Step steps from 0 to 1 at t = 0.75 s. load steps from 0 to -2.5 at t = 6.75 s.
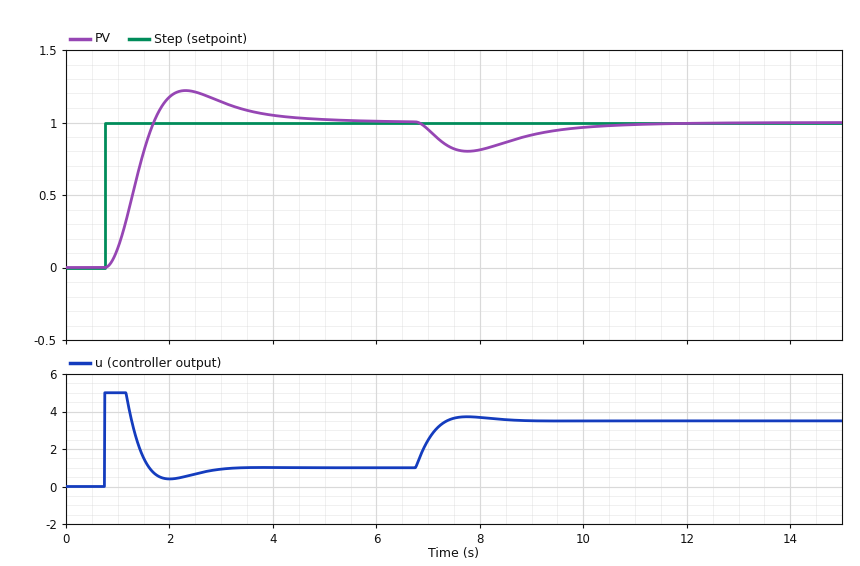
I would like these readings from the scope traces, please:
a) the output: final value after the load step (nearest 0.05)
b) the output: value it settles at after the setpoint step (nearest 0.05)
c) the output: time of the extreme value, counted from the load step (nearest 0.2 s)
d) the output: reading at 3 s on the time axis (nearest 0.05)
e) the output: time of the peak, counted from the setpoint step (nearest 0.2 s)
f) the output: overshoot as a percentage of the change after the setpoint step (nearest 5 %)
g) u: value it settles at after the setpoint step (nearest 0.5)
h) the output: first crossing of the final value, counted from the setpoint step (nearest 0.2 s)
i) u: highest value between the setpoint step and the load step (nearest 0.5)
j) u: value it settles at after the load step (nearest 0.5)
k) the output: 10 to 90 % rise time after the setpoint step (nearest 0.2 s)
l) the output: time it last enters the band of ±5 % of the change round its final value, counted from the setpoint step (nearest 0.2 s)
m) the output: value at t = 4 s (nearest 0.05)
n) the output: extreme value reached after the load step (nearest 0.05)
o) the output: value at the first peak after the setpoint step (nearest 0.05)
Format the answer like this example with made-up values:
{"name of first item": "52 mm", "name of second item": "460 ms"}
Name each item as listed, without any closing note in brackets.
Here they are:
{"the output: final value after the load step": "1.00", "the output: value it settles at after the setpoint step": "1.00", "the output: time of the extreme value, counted from the load step": "1.0 s", "the output: reading at 3 s on the time axis": "1.15", "the output: time of the peak, counted from the setpoint step": "1.6 s", "the output: overshoot as a percentage of the change after the setpoint step": "20 %", "u: value it settles at after the setpoint step": "1.0", "the output: first crossing of the final value, counted from the setpoint step": "1.0 s", "u: highest value between the setpoint step and the load step": "5.0", "u: value it settles at after the load step": "3.5", "the output: 10 to 90 % rise time after the setpoint step": "0.6 s", "the output: time it last enters the band of ±5 % of the change round its final value, counted from the setpoint step": "3.2 s", "the output: value at t = 4 s": "1.05", "the output: extreme value reached after the load step": "0.80", "the output: value at the first peak after the setpoint step": "1.20"}
